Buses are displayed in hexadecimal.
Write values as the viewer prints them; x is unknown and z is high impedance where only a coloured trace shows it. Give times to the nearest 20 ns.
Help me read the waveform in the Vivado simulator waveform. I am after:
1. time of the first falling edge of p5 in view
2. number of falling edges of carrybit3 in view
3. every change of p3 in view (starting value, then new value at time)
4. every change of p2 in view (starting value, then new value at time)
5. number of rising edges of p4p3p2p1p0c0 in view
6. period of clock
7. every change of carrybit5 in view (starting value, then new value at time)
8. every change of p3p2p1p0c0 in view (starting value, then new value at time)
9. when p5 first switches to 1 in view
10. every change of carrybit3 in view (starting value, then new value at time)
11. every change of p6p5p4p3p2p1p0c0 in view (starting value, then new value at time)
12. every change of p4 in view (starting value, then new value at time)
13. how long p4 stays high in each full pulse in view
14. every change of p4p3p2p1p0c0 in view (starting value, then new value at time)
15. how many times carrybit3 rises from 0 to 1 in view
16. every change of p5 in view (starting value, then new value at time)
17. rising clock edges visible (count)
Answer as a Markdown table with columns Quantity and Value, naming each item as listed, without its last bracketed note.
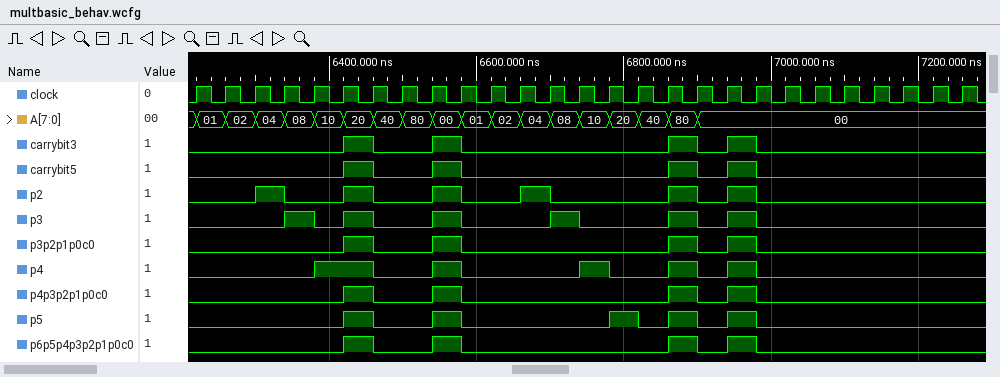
| Quantity | Value |
|---|---|
| time of the first falling edge of p5 in view | 6460 ns |
| number of falling edges of carrybit3 in view | 4 |
| every change of p3 in view | 0, 1 at 6340 ns, 0 at 6380 ns, 1 at 6420 ns, 0 at 6460 ns, 1 at 6540 ns, 0 at 6580 ns, 1 at 6700 ns, 0 at 6740 ns, 1 at 6860 ns, 0 at 6900 ns, 1 at 6940 ns, 0 at 6980 ns |
| every change of p2 in view | 0, 1 at 6300 ns, 0 at 6340 ns, 1 at 6420 ns, 0 at 6460 ns, 1 at 6540 ns, 0 at 6580 ns, 1 at 6660 ns, 0 at 6700 ns, 1 at 6860 ns, 0 at 6900 ns, 1 at 6940 ns, 0 at 6980 ns |
| number of rising edges of p4p3p2p1p0c0 in view | 4 |
| period of clock | 40 ns |
| every change of carrybit5 in view | 0, 1 at 6420 ns, 0 at 6460 ns, 1 at 6540 ns, 0 at 6580 ns, 1 at 6860 ns, 0 at 6900 ns, 1 at 6940 ns, 0 at 6980 ns |
| every change of p3p2p1p0c0 in view | 0, 1 at 6420 ns, 0 at 6460 ns, 1 at 6540 ns, 0 at 6580 ns, 1 at 6860 ns, 0 at 6900 ns, 1 at 6940 ns, 0 at 6980 ns |
| when p5 first switches to 1 in view | 6420 ns |
| every change of carrybit3 in view | 0, 1 at 6420 ns, 0 at 6460 ns, 1 at 6540 ns, 0 at 6580 ns, 1 at 6860 ns, 0 at 6900 ns, 1 at 6940 ns, 0 at 6980 ns |
| every change of p6p5p4p3p2p1p0c0 in view | 0, 1 at 6420 ns, 0 at 6460 ns, 1 at 6540 ns, 0 at 6580 ns, 1 at 6860 ns, 0 at 6900 ns, 1 at 6940 ns, 0 at 6980 ns |
| every change of p4 in view | 0, 1 at 6380 ns, 0 at 6460 ns, 1 at 6540 ns, 0 at 6580 ns, 1 at 6740 ns, 0 at 6780 ns, 1 at 6860 ns, 0 at 6900 ns, 1 at 6940 ns, 0 at 6980 ns |
| how long p4 stays high in each full pulse in view | 80 ns, 40 ns, 40 ns, 40 ns, 40 ns |
| every change of p4p3p2p1p0c0 in view | 0, 1 at 6420 ns, 0 at 6460 ns, 1 at 6540 ns, 0 at 6580 ns, 1 at 6860 ns, 0 at 6900 ns, 1 at 6940 ns, 0 at 6980 ns |
| how many times carrybit3 rises from 0 to 1 in view | 4 |
| every change of p5 in view | 0, 1 at 6420 ns, 0 at 6460 ns, 1 at 6540 ns, 0 at 6580 ns, 1 at 6780 ns, 0 at 6820 ns, 1 at 6860 ns, 0 at 6900 ns, 1 at 6940 ns, 0 at 6980 ns |
| rising clock edges visible | 27 |
